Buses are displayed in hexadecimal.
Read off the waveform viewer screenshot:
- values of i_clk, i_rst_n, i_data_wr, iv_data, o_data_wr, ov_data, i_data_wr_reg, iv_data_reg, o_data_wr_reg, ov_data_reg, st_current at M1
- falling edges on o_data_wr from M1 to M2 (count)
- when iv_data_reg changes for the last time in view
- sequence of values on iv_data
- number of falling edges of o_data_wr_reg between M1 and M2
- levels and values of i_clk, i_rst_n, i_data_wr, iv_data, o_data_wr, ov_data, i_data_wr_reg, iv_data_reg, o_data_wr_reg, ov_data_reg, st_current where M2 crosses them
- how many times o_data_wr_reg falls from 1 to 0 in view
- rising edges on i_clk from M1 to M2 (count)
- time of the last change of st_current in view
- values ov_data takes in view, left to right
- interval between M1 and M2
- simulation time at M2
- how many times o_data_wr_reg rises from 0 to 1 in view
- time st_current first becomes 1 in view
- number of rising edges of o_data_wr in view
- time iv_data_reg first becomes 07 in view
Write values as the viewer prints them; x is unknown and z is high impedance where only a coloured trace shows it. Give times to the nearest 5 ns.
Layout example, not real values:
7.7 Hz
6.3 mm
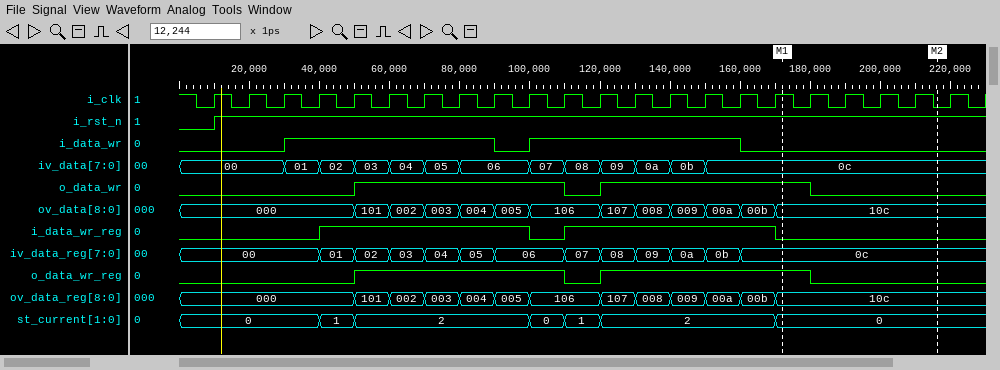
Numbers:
i_clk=1, i_rst_n=1, i_data_wr=0, iv_data=0c, o_data_wr=1, ov_data=10c, i_data_wr_reg=0, iv_data_reg=0c, o_data_wr_reg=1, ov_data_reg=10c, st_current=0
1
160 ns
00, 01, 02, 03, 04, 05, 06, 07, 08, 09, 0a, 0b, 0c
1
i_clk=0, i_rst_n=1, i_data_wr=0, iv_data=0c, o_data_wr=0, ov_data=10c, i_data_wr_reg=0, iv_data_reg=0c, o_data_wr_reg=0, ov_data_reg=10c, st_current=0
2
4
170 ns
000, 101, 002, 003, 004, 005, 106, 107, 008, 009, 00a, 00b, 10c
45 ns
215 ns
2
40 ns
2
110 ns
